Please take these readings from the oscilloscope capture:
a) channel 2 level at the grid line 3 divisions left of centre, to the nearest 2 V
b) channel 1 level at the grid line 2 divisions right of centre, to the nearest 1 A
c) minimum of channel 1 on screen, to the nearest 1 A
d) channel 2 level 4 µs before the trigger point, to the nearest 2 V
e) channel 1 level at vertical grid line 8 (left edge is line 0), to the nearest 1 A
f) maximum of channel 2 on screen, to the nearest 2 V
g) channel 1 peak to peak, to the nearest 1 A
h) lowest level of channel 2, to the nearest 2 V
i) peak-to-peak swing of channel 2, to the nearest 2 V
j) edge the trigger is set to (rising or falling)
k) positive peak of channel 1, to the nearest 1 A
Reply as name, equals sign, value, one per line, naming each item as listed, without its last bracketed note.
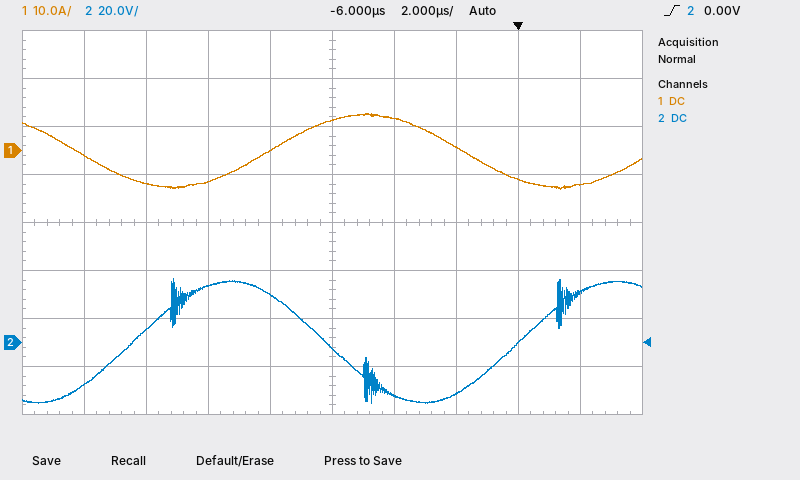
channel 2 level at the grid line 3 divisions left of centre, to the nearest 2 V = 6 V
channel 1 level at the grid line 2 divisions right of centre, to the nearest 1 A = 1 A
minimum of channel 1 on screen, to the nearest 1 A = -8 A
channel 2 level 4 µs before the trigger point, to the nearest 2 V = -22 V
channel 1 level at vertical grid line 8 (left edge is line 0), to the nearest 1 A = -6 A
maximum of channel 2 on screen, to the nearest 2 V = 26 V
channel 1 peak to peak, to the nearest 1 A = 16 A
lowest level of channel 2, to the nearest 2 V = -26 V
peak-to-peak swing of channel 2, to the nearest 2 V = 52 V
edge the trigger is set to = rising
positive peak of channel 1, to the nearest 1 A = 8 A
